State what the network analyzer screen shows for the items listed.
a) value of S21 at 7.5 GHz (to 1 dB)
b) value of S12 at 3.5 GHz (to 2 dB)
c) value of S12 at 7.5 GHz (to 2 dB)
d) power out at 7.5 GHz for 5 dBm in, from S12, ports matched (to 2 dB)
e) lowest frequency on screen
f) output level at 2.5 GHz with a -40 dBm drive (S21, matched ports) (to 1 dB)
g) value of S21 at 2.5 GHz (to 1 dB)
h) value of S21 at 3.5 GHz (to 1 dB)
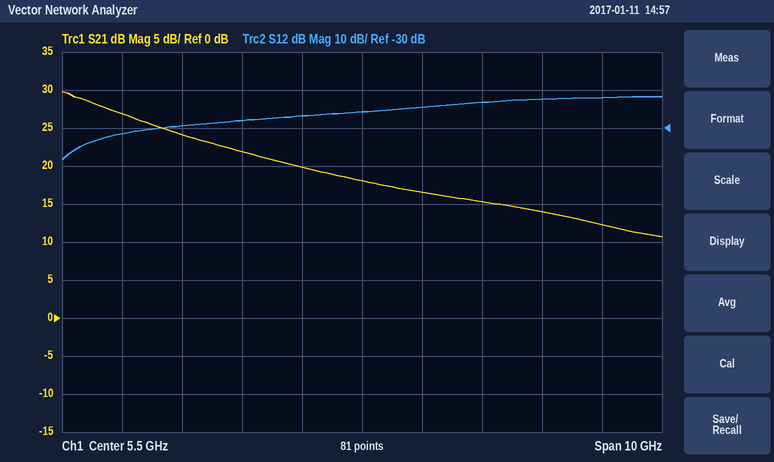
15 dB
-28 dB
-24 dB
-18 dBm
500 MHz
-16 dBm
24 dB
22 dB
